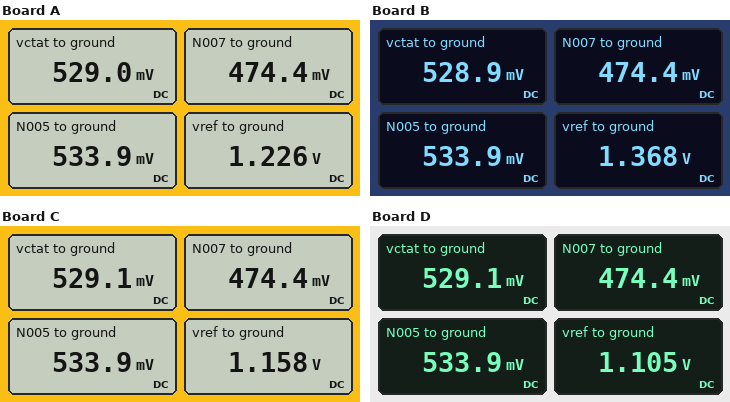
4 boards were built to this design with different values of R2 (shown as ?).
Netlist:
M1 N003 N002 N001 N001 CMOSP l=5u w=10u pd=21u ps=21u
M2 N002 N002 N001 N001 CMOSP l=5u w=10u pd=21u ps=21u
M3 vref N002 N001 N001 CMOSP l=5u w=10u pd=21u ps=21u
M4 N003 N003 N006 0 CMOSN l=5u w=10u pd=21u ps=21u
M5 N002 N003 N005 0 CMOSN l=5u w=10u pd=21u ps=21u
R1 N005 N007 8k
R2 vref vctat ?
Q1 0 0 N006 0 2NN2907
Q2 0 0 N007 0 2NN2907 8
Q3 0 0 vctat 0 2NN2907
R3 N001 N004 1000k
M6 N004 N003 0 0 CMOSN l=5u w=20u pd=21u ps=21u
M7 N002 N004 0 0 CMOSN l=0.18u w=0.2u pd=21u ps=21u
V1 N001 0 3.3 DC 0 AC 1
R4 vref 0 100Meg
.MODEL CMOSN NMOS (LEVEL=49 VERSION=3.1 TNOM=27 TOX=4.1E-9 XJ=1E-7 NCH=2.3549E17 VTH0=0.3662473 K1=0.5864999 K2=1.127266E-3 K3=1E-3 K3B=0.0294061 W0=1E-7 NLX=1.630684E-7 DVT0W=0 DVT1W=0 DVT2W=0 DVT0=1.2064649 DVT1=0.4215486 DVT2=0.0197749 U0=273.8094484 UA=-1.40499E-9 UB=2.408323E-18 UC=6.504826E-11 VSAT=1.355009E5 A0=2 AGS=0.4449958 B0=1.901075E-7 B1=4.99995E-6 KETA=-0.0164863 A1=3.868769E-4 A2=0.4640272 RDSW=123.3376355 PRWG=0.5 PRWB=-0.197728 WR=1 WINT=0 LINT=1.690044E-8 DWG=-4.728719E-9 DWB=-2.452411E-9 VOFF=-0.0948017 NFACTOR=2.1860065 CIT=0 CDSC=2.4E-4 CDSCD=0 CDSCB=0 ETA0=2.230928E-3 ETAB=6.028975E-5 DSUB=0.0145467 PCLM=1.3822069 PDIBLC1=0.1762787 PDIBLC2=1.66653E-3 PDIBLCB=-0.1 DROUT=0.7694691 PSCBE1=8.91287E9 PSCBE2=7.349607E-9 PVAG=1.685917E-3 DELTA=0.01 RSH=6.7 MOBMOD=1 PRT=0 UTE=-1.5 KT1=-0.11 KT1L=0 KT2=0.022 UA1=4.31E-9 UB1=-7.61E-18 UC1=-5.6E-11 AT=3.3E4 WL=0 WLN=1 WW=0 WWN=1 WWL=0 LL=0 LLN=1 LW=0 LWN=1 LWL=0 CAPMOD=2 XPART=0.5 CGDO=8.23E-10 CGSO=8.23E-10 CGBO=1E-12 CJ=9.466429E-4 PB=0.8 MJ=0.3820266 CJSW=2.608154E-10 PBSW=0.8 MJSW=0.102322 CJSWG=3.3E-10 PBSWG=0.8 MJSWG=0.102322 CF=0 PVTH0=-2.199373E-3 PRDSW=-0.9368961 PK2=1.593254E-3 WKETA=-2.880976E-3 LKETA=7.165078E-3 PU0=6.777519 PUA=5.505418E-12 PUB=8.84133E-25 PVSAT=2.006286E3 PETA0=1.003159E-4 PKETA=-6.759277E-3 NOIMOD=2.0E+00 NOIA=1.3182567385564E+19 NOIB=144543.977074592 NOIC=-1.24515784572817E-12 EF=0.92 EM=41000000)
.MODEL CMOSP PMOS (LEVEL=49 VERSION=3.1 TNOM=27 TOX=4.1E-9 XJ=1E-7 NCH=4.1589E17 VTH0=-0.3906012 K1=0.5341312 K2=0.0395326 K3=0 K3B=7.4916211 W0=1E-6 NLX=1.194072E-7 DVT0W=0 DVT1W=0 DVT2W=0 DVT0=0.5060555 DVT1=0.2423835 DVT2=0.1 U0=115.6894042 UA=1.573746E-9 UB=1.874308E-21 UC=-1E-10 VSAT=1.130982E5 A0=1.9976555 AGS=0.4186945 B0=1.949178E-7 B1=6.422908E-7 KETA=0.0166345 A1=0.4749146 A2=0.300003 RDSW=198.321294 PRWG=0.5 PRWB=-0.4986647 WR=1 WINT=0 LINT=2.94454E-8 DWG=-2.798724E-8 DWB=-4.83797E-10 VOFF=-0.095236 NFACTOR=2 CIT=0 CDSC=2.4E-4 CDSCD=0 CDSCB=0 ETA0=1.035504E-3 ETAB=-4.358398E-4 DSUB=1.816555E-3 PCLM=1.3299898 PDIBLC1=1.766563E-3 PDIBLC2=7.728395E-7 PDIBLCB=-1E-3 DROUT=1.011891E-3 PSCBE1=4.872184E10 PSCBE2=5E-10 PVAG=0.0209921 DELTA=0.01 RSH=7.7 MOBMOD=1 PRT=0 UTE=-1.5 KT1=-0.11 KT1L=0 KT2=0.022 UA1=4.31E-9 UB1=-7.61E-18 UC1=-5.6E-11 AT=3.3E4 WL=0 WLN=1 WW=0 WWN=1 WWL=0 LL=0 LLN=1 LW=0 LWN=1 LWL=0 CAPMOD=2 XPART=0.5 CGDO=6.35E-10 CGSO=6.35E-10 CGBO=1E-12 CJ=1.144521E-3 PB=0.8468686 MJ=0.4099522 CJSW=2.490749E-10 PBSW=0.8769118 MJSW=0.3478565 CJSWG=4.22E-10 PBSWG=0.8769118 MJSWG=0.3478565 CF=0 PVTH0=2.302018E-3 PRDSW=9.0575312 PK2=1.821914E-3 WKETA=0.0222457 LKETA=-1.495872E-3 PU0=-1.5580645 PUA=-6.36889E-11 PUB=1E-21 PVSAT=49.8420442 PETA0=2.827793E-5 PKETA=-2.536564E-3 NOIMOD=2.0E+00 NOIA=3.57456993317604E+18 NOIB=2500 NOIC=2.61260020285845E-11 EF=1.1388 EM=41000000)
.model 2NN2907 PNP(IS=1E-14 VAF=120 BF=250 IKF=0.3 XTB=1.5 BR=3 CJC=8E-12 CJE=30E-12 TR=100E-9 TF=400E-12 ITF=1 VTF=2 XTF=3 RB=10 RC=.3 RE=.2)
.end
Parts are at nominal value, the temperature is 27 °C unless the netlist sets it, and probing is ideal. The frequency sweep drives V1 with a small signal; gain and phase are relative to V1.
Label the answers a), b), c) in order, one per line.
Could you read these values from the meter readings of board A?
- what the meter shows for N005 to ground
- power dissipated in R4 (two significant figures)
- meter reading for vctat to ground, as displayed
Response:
a) 533.9 mV
b) 15 nW
c) 529.0 mV
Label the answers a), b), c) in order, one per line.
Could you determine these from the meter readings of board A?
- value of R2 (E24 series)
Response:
a) 91 kΩ
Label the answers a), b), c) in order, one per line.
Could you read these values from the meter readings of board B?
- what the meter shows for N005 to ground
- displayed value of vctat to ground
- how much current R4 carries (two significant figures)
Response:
a) 533.9 mV
b) 528.9 mV
c) 14 nA
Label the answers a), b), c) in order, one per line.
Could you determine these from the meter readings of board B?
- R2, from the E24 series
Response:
a) 110 kΩ
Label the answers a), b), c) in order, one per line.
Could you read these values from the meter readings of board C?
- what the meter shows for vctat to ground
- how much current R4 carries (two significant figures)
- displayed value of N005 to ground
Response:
a) 529.1 mV
b) 12 nA
c) 533.9 mV
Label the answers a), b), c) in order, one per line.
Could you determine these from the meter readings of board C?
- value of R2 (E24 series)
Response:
a) 82 kΩ
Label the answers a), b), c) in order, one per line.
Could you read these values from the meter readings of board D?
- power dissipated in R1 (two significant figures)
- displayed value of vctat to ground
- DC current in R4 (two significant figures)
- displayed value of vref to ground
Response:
a) 440 nW
b) 529.1 mV
c) 11 nA
d) 1.105 V
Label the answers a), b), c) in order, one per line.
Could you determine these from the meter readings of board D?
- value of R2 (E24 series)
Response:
a) 75 kΩ
